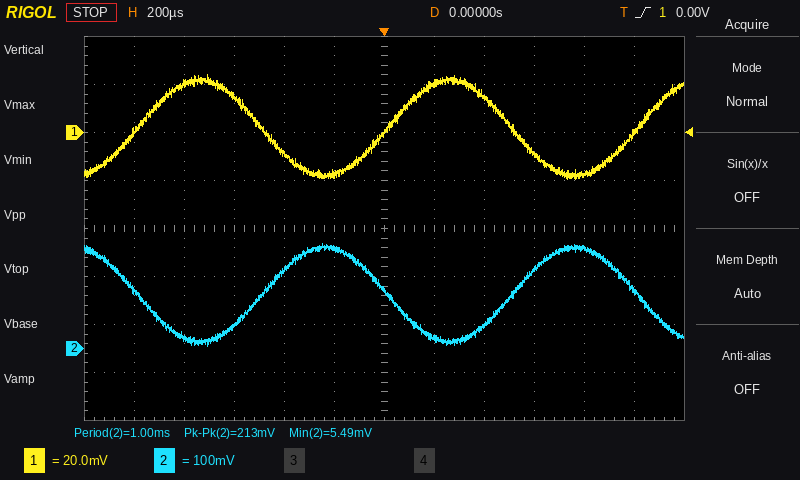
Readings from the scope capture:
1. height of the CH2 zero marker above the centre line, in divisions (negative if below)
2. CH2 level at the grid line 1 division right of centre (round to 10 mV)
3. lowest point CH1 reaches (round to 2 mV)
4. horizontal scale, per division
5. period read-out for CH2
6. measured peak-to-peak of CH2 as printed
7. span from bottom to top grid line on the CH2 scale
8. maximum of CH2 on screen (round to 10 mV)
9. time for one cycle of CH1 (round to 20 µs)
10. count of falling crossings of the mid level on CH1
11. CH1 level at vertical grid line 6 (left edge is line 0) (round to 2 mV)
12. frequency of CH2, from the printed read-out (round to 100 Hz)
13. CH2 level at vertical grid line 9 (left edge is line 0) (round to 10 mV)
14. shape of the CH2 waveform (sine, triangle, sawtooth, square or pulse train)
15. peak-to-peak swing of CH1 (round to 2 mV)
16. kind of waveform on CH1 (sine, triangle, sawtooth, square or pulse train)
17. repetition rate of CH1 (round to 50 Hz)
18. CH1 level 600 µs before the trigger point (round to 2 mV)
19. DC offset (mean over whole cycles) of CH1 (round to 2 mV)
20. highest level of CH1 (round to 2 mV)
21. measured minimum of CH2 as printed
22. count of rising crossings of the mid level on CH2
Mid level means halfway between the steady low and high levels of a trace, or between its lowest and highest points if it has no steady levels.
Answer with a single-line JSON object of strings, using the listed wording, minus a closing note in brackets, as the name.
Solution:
{"height of the CH2 zero marker above the centre line, in divisions": "-2.5 div", "CH2 level at the grid line 1 division right of centre": "20 mV", "lowest point CH1 reaches": "-20 mV", "horizontal scale, per division": "200 µs", "period read-out for CH2": "1.00 ms", "measured peak-to-peak of CH2 as printed": "213 mV", "span from bottom to top grid line on the CH2 scale": "800 mV", "maximum of CH2 on screen": "220 mV", "time for one cycle of CH1": "1.00 ms", "count of falling crossings of the mid level on CH1": "2", "CH1 level at vertical grid line 6 (left edge is line 0)": "0 mV", "frequency of CH2, from the printed read-out": "1.0 kHz", "CH2 level at vertical grid line 9 (left edge is line 0)": "160 mV", "shape of the CH2 waveform": "sine", "peak-to-peak swing of CH1": "44 mV", "kind of waveform on CH1": "sine", "repetition rate of CH1": "1.00 kHz", "CH1 level 600 µs before the trigger point": "16 mV", "DC offset (mean over whole cycles) of CH1": "2 mV", "highest level of CH1": "24 mV", "measured minimum of CH2 as printed": "5.49 mV", "count of rising crossings of the mid level on CH2": "2"}
